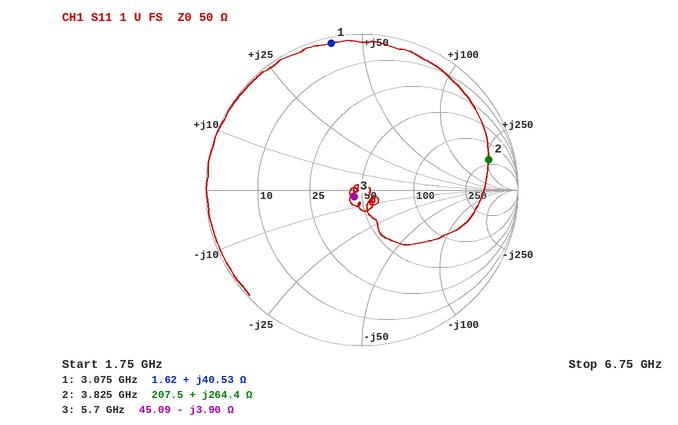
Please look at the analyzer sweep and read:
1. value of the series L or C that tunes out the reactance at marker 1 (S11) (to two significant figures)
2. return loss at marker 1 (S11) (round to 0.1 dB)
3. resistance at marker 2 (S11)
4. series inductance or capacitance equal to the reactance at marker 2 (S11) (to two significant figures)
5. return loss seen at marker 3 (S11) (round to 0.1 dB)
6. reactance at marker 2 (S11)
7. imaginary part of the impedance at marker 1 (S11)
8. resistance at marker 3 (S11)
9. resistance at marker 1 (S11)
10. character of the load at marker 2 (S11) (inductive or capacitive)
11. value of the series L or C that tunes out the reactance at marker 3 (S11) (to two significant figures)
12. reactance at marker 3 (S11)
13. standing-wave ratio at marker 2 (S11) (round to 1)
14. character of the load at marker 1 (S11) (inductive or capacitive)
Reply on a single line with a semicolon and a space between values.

1.3 pF; 0.3 dB; 207.5 Ω; 11 nH; 23.6 dB; +264.4 Ω; +40.53 Ω; 45.09 Ω; 1.62 Ω; inductive; 110 pH; -3.90 Ω; 11; inductive
